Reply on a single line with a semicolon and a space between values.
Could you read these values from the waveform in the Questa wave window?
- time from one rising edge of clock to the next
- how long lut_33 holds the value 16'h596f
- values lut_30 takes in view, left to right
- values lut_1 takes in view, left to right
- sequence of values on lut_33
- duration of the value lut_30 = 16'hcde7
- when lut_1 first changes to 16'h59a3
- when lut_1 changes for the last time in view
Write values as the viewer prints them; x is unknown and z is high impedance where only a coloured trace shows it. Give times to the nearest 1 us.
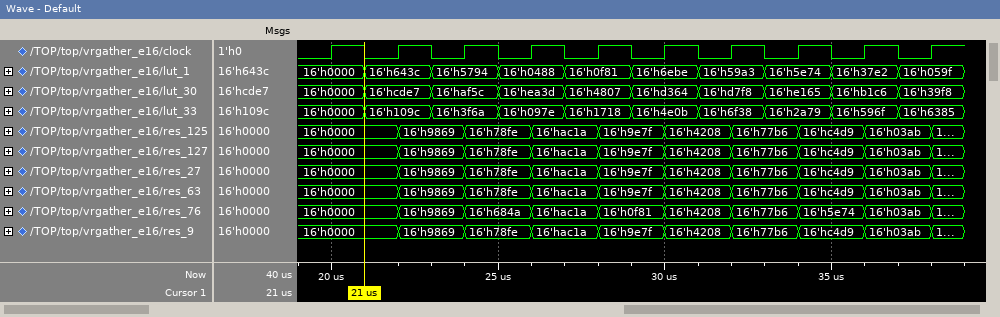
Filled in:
2 us; 2 us; 16'h0000, 16'hcde7, 16'haf5c, 16'hea3d, 16'h4807, 16'hd364, 16'hd7f8, 16'he165, 16'hb1c6, 16'h39f8; 16'h0000, 16'h643c, 16'h5794, 16'h0488, 16'h0f81, 16'h6ebe, 16'h59a3, 16'h5e74, 16'h37e2, 16'h059f; 16'h0000, 16'h109c, 16'h3f6a, 16'h097e, 16'h1718, 16'h4e0b, 16'h6f38, 16'h2a79, 16'h596f, 16'h6385; 2 us; 31 us; 37 us
